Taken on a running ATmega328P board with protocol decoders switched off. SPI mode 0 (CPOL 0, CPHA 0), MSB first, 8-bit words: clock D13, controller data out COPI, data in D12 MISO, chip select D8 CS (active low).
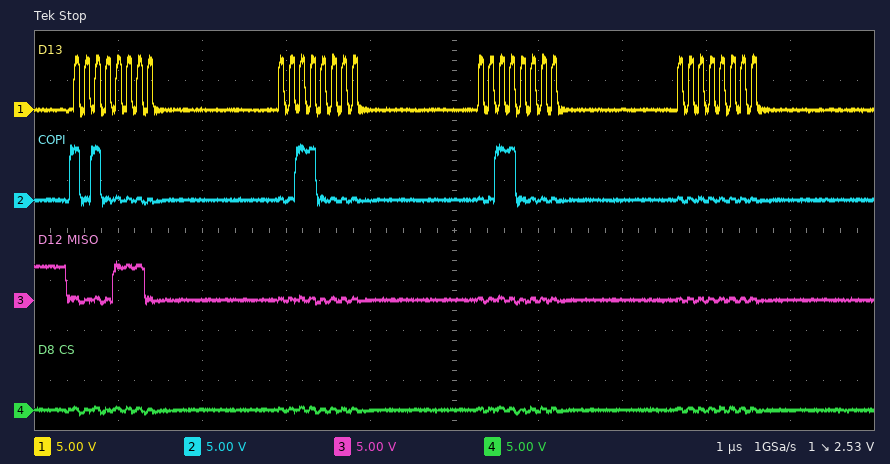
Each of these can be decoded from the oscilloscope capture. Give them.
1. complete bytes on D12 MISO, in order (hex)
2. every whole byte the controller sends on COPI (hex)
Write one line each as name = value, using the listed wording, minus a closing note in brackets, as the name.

complete bytes on D12 MISO, in order = 0E 00 00 00
every whole byte the controller sends on COPI = A0 30 30 00
